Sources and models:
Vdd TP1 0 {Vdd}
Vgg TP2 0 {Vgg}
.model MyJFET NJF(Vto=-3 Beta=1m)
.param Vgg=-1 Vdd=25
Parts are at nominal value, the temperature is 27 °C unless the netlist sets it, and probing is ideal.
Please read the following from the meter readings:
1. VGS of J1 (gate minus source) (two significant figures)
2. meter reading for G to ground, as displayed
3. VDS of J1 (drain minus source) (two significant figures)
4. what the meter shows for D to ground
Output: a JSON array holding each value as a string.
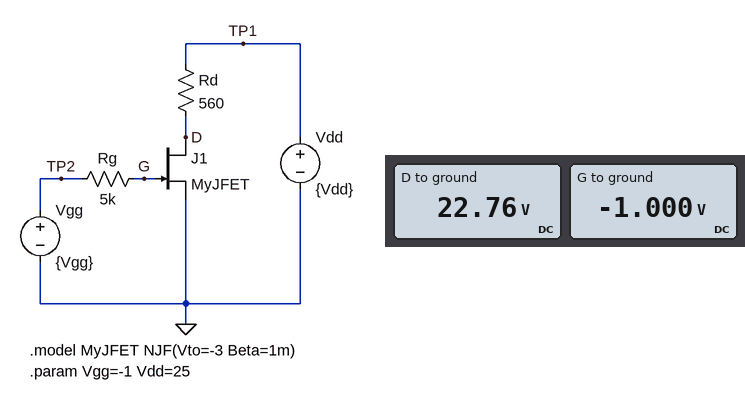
["-1.0 V", "-1.000 V", "23 V", "22.76 V"]
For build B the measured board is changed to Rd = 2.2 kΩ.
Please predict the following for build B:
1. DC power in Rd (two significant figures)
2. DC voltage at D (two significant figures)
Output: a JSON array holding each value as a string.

["35 mW", "16 V"]
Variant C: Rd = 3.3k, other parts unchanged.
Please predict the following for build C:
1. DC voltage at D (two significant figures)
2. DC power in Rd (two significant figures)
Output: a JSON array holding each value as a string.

["12 V", "53 mW"]
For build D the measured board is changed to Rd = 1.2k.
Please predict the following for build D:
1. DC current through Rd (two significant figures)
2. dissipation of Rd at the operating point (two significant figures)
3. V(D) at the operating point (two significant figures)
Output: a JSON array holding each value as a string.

["4.0 mA", "19 mW", "20 V"]
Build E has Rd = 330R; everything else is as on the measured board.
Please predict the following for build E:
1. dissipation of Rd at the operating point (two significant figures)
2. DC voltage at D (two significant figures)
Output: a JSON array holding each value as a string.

["5.3 mW", "24 V"]
